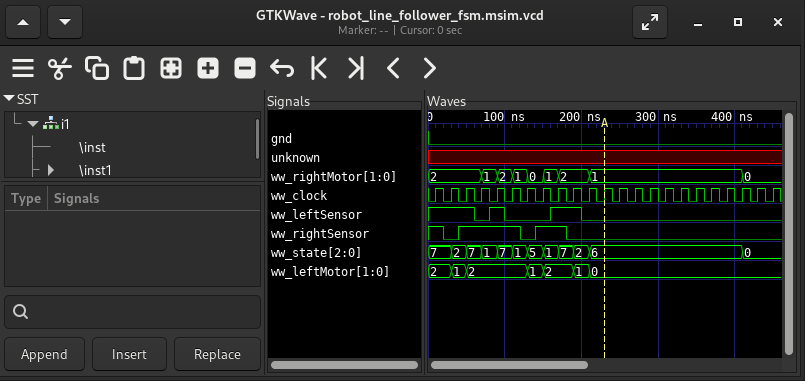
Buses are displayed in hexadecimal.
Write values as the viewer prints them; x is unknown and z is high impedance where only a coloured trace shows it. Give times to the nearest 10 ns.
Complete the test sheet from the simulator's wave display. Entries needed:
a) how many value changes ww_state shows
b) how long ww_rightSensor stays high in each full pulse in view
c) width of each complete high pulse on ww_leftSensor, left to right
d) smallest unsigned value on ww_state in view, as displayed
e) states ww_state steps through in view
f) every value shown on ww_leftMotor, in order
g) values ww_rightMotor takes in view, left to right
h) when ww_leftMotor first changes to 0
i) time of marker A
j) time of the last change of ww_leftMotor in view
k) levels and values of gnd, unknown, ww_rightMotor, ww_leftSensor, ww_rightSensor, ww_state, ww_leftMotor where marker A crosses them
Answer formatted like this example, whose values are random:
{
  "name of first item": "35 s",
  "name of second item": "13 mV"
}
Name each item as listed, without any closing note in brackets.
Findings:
{
  "how many value changes ww_state shows": "11",
  "how long ww_rightSensor stays high in each full pulse in view": "80 ns, 40 ns",
  "width of each complete high pulse on ww_leftSensor, left to right": "20 ns, 40 ns",
  "smallest unsigned value on ww_state in view, as displayed": "0",
  "states ww_state steps through in view": "7, 2, 7, 1, 7, 1, 5, 1, 7, 2, 6, 0",
  "every value shown on ww_leftMotor, in order": "2, 1, 2, 1, 2, 1, 0",
  "values ww_rightMotor takes in view, left to right": "2, 1, 2, 1, 0, 1, 2, 1, 0",
  "when ww_leftMotor first changes to 0": "210 ns",
  "time of marker A": "230 ns",
  "time of the last change of ww_leftMotor in view": "210 ns",
  "levels and values of gnd, unknown, ww_rightMotor, ww_leftSensor, ww_rightSensor, ww_state, ww_leftMotor where marker A crosses them": "gnd=0, unknown=x, ww_rightMotor=1, ww_leftSensor=0, ww_rightSensor=0, ww_state=6, ww_leftMotor=0"
}
